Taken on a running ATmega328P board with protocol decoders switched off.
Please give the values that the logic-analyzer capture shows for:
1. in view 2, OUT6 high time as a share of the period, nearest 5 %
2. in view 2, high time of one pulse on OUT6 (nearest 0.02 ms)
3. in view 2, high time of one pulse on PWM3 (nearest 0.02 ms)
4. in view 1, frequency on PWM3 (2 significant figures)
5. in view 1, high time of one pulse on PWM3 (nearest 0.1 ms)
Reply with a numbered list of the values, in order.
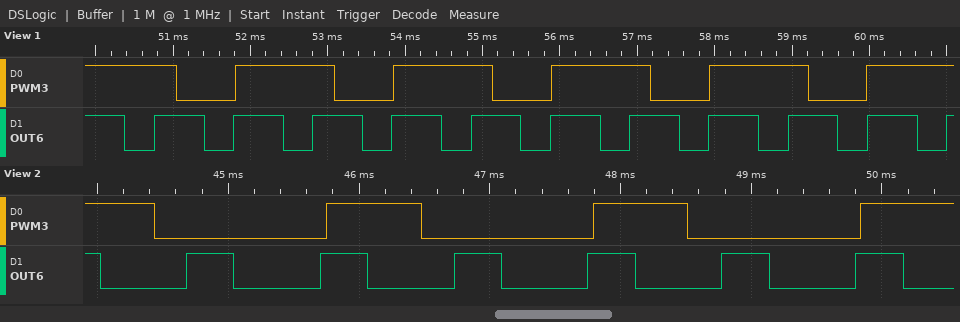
1. 35 %
2. 0.36 ms
3. 0.72 ms
4. 490 Hz
5. 1.3 ms
